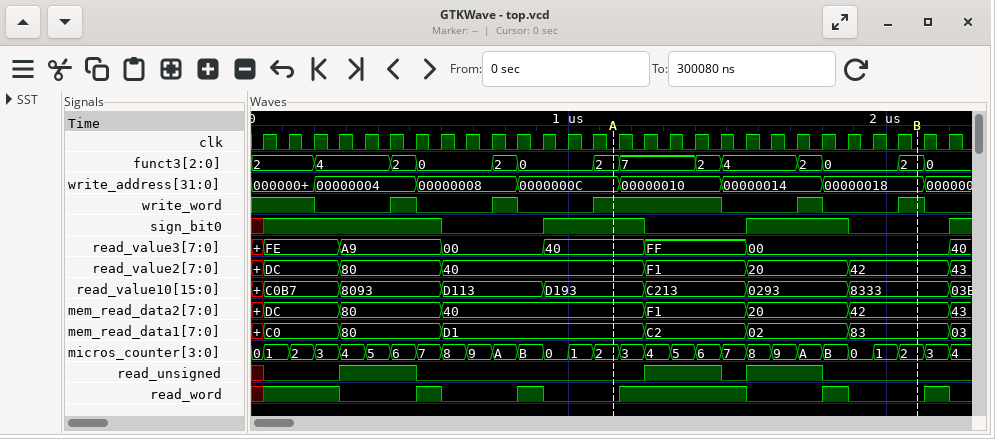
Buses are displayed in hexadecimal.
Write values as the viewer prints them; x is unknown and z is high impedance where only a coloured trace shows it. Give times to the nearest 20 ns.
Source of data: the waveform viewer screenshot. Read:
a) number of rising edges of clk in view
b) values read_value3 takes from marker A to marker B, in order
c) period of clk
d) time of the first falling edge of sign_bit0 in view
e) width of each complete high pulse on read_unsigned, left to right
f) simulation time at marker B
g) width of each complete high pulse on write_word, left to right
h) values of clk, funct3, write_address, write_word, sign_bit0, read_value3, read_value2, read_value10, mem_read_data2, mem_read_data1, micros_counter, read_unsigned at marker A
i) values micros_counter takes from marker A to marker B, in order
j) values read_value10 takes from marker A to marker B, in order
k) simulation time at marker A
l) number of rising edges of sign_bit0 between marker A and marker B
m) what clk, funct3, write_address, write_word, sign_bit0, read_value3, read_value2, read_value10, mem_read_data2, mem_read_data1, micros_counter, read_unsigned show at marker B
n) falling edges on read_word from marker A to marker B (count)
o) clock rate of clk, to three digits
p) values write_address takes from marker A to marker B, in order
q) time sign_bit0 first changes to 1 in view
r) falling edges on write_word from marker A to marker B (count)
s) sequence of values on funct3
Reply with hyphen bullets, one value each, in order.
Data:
- 28
- 40, FF, 00
- 80 ns
- 600 ns
- 240 ns, 240 ns, 240 ns
- 2100 ns
- 80 ns, 80 ns, 400 ns, 80 ns, 80 ns
- clk=0, funct3=2, write_address=0000000C, write_word=1, sign_bit0=1, read_value3=40, read_value2=40, read_value10=D193, mem_read_data2=40, mem_read_data1=D1, micros_counter=2, read_unsigned=0
- 2, 3, 4, 5, 6, 7, 8, 9, A, B, 0, 1, 2
- D193, C213, 0293, 8333
- 1140 ns
- 1
- clk=0, funct3=2, write_address=00000018, write_word=1, sign_bit0=0, read_value3=00, read_value2=42, read_value10=8333, mem_read_data2=42, mem_read_data1=83, micros_counter=2, read_unsigned=0
- 2
- 12.5 MHz
- 0000000C, 00000010, 00000014, 00000018
- 40 ns
- 2
- 2, 4, 2, 0, 2, 0, 2, 7, 2, 4, 2, 0, 2, 0
